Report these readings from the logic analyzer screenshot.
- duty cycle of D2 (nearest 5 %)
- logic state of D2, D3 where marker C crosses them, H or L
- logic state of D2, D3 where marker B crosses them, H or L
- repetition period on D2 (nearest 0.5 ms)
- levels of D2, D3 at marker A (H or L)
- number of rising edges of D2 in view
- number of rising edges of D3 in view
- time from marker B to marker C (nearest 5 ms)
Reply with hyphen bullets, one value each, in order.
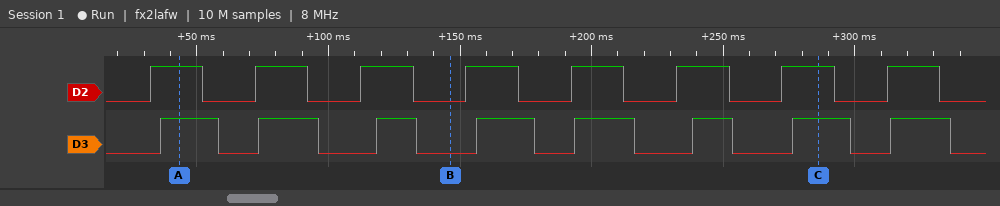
- 50 %
- D2=H, D3=H
- D2=L, D3=L
- 40 ms
- D2=H, D3=H
- 8
- 8
- 140 ms
